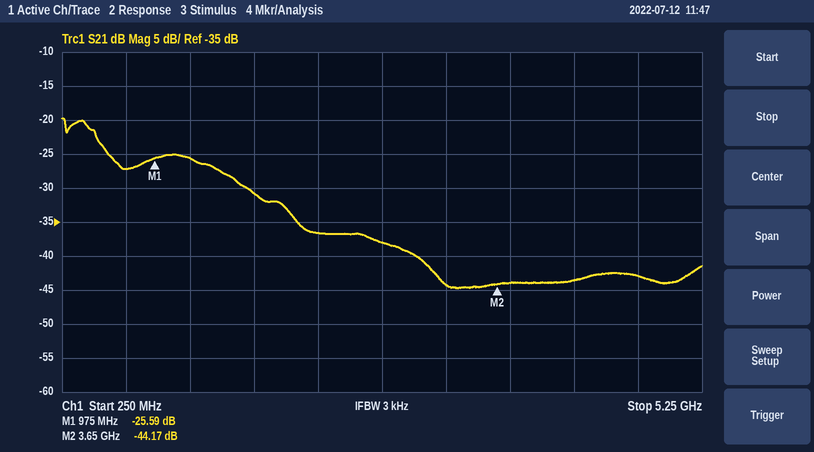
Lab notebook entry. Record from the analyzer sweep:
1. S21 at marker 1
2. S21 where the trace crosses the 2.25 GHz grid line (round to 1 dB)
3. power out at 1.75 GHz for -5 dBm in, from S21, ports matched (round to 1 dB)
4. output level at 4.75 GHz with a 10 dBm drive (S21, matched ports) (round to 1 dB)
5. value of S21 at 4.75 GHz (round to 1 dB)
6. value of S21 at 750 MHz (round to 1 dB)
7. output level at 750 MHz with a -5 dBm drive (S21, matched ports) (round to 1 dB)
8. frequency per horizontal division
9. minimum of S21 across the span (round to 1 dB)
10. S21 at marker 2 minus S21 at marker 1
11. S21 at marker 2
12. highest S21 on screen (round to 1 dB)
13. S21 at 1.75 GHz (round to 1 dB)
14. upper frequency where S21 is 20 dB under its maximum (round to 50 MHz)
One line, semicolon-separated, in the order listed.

-25.59 dB; -37 dB; -36 dBm; -33 dBm; -43 dB; -27 dB; -32 dBm; 500 MHz; -45 dB; -18.58 dB; -44.17 dB; -20 dB; -31 dB; 3.00 GHz
